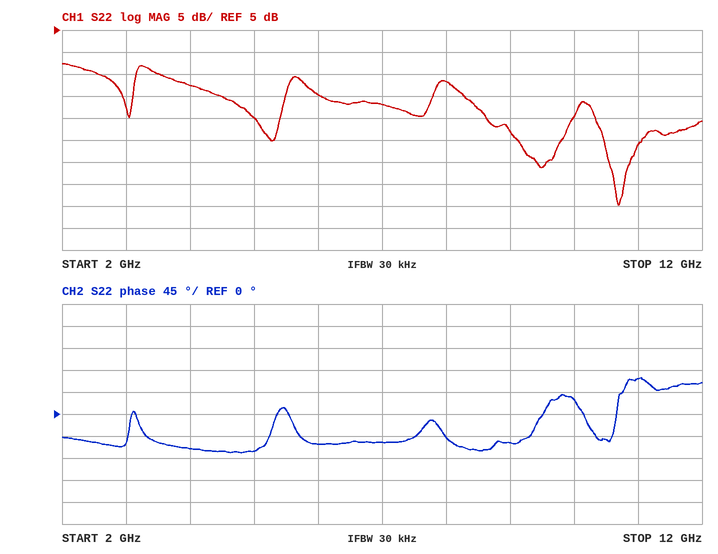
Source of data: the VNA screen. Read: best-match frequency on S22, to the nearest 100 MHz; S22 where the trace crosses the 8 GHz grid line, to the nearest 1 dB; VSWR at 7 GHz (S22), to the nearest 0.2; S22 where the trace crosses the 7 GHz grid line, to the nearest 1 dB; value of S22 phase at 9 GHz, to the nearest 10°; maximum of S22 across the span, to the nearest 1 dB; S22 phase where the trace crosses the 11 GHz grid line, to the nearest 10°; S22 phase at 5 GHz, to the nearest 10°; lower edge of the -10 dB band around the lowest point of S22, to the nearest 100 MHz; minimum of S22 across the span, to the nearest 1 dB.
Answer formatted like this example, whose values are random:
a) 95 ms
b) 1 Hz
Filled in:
a) 10.7 GHz
b) -7 dB
c) 1.6
d) -12 dB
e) -60°
f) -3 dB
g) 70°
h) -80°
i) 8.3 GHz
j) -35 dB
